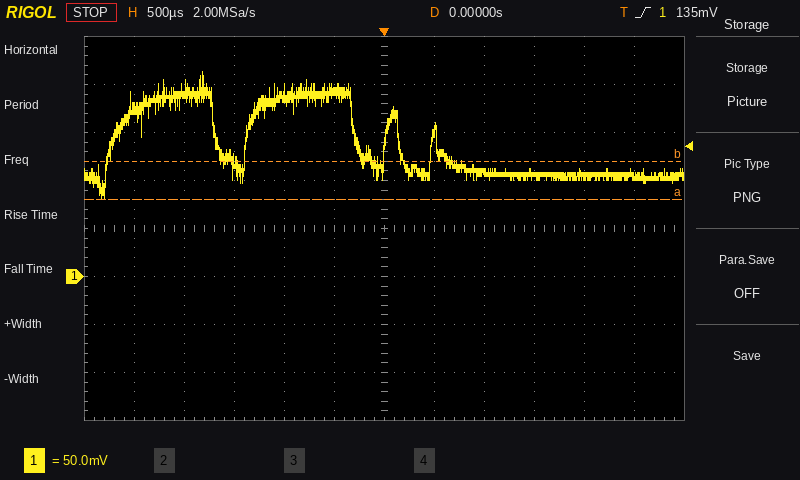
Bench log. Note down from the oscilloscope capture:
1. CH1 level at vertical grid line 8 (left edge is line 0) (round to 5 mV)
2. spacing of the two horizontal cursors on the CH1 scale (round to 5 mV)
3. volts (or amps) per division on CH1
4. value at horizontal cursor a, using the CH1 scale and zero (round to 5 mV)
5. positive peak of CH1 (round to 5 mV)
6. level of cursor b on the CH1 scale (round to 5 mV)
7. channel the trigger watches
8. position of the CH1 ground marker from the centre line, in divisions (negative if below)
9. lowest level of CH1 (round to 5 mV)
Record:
110 mV
40 mV
50 mV
80 mV
215 mV
120 mV
CH1
-1.0 div
80 mV
